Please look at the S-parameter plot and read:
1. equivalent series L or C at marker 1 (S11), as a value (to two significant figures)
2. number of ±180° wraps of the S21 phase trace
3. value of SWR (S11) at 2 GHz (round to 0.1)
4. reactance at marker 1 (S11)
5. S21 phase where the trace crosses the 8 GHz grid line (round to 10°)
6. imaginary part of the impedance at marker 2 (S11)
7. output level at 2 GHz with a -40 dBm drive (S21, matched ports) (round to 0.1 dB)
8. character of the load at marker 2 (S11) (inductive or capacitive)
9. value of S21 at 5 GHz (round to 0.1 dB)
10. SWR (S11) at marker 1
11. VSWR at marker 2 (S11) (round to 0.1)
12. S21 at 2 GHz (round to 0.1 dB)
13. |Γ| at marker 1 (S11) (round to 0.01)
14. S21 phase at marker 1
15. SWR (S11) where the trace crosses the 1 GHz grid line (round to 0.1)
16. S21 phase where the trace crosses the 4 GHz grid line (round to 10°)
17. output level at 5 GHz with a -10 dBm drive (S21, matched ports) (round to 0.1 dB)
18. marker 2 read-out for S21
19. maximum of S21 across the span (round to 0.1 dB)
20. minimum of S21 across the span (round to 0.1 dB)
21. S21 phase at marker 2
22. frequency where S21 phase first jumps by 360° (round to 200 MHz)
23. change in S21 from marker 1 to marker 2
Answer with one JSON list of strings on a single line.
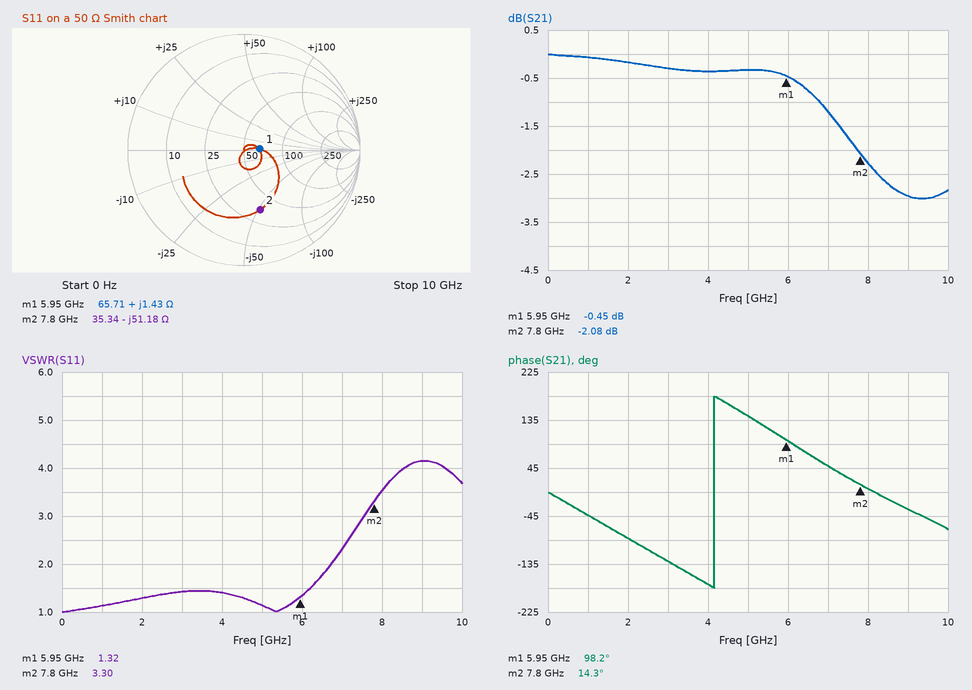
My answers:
["38 pH", "1", "1.3", "+1.43 Ω", "10°", "-51.18 Ω", "-40.2 dBm", "capacitive", "-0.3 dB", "1.32", "3.3", "-0.2 dB", "0.14", "98.2°", "1.1", "-170°", "-10.3 dBm", "-2.08 dB", "0.0 dB", "-3.0 dB", "14.3°", "4.2 GHz", "-1.63 dB"]
